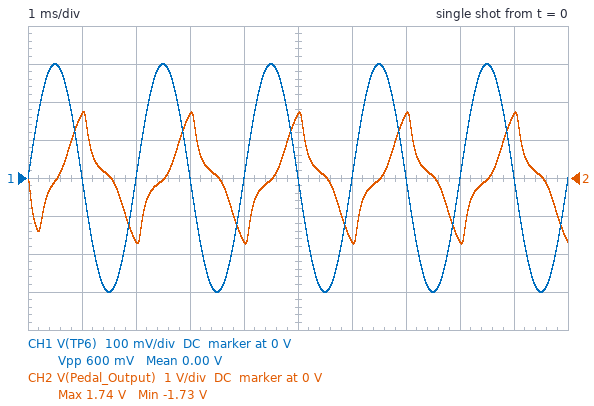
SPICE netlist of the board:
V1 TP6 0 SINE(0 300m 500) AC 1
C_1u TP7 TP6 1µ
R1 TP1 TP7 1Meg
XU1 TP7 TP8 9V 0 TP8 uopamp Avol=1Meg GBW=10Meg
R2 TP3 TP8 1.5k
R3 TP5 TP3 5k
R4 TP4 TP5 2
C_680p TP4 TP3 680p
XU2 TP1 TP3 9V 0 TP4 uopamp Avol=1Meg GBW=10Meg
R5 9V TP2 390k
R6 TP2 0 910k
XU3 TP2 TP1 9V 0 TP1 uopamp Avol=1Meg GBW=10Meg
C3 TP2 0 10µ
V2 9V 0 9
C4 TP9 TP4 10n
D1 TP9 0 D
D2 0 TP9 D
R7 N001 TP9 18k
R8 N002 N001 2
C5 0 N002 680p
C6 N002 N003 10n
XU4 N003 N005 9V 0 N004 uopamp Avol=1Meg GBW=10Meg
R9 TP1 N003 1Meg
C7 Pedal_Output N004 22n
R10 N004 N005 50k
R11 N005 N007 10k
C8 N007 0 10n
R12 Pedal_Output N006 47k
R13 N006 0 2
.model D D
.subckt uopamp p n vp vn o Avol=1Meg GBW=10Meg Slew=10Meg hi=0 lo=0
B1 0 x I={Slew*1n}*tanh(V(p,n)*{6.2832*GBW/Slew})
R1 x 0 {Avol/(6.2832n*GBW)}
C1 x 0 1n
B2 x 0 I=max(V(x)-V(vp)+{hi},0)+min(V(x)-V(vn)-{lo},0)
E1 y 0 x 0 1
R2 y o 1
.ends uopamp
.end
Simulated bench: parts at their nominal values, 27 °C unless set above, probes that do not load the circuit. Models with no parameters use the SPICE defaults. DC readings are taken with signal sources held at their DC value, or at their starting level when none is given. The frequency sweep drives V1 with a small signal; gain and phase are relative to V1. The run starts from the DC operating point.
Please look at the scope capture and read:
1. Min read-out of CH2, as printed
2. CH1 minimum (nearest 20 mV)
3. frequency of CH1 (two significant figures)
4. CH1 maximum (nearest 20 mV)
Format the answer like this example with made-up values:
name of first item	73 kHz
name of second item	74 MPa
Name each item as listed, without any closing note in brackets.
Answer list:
Min read-out of CH2, as printed	-1.73 V
CH1 minimum	-300 mV
frequency of CH1	500 Hz
CH1 maximum	300 mV
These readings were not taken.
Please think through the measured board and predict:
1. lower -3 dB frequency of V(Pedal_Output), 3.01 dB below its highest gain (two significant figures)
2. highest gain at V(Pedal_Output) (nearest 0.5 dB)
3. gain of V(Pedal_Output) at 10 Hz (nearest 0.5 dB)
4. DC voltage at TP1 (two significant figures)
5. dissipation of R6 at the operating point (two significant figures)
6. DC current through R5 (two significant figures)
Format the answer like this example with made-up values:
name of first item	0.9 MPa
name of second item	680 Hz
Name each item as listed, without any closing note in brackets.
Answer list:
lower -3 dB frequency of V(Pedal_Output), 3.01 dB below its highest gain	1.3 kHz
highest gain at V(Pedal_Output)	24.5 dB
gain of V(Pedal_Output) at 10 Hz	-24.0 dB
DC voltage at TP1	6.3 V
dissipation of R6 at the operating point	44 µW
DC current through R5	6.9 µA
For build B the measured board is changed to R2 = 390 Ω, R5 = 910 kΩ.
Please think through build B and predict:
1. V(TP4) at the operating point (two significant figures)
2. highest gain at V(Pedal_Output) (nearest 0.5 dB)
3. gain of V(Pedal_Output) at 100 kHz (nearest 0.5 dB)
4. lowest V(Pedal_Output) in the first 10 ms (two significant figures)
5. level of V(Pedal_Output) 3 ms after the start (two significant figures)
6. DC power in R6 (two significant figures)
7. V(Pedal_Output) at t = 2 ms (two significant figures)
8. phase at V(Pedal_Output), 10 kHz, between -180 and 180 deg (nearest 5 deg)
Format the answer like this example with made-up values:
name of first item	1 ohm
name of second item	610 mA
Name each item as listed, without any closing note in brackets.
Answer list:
V(TP4) at the operating point	4.5 V
highest gain at V(Pedal_Output)	36.0 dB
gain of V(Pedal_Output) at 100 kHz	12.0 dB
lowest V(Pedal_Output) in the first 10 ms	-3.1 V
level of V(Pedal_Output) 3 ms after the start	570 mV
DC power in R6	22 µW
V(Pedal_Output) at t = 2 ms	-570 mV
phase at V(Pedal_Output), 10 kHz, between -180 and 180 deg	140 deg
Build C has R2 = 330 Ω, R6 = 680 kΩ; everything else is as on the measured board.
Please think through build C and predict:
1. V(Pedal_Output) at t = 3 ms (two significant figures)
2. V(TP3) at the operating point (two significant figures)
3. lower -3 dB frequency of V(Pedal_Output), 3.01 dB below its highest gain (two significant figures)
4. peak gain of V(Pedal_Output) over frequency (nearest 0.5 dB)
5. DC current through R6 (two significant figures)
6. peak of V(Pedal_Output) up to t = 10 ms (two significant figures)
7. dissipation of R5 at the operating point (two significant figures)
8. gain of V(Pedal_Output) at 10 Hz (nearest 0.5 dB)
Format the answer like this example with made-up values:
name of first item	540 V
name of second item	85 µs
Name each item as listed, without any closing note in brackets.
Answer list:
V(Pedal_Output) at t = 3 ms	510 mV
V(TP3) at the operating point	5.7 V
lower -3 dB frequency of V(Pedal_Output), 3.01 dB below its highest gain	1.3 kHz
peak gain of V(Pedal_Output) over frequency	37.5 dB
DC current through R6	8.4 µA
peak of V(Pedal_Output) up to t = 10 ms	3.3 V
dissipation of R5 at the operating point	28 µW
gain of V(Pedal_Output) at 10 Hz	-11.0 dB
